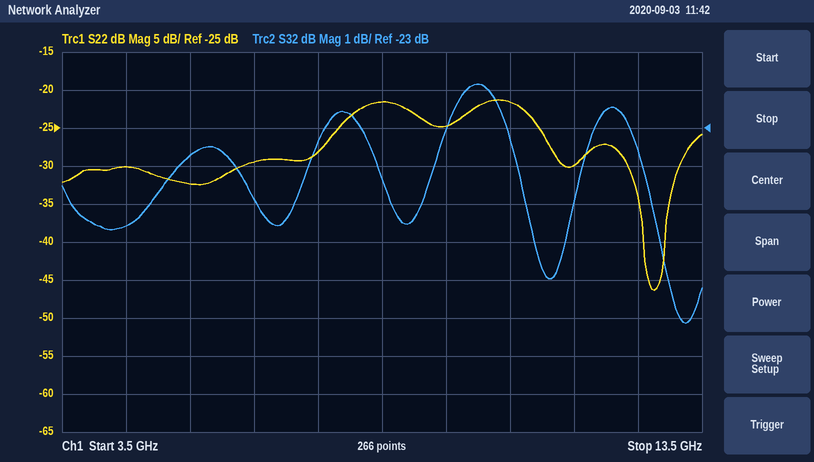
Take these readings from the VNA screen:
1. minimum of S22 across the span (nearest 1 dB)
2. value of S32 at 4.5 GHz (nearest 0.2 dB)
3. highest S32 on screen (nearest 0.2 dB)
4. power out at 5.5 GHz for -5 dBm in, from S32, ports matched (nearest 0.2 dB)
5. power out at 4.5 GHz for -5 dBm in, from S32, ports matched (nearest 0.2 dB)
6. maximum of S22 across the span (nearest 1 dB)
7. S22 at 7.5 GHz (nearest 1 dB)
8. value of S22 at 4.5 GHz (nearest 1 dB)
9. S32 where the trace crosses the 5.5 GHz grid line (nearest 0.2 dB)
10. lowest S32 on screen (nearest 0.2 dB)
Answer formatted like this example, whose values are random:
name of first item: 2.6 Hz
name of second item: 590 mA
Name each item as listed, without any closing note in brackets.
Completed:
minimum of S22 across the span: -46 dB
value of S32 at 4.5 GHz: -25.6 dB
highest S32 on screen: -21.8 dB
power out at 5.5 GHz for -5 dBm in, from S32, ports matched: -28.8 dBm
power out at 4.5 GHz for -5 dBm in, from S32, ports matched: -30.6 dBm
maximum of S22 across the span: -21 dB
S22 at 7.5 GHz: -28 dB
value of S22 at 4.5 GHz: -30 dB
S32 where the trace crosses the 5.5 GHz grid line: -23.8 dB
lowest S32 on screen: -28.2 dB
